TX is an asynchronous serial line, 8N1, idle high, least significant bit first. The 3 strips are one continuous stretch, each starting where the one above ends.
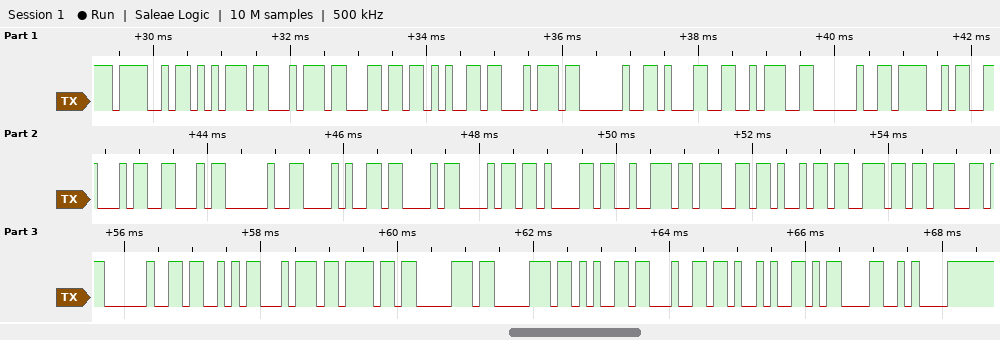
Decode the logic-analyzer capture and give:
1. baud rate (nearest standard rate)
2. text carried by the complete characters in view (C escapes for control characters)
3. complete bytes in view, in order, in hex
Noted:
9600 baud
"Outlet 1: OFF (Charging Stopped)\r\n"
0x4F 0x75 0x74 0x6C 0x65 0x74 0x20 0x31 0x3A 0x20 0x4F 0x46 0x46 0x20 0x28 0x43 0x68 0x61 0x72 0x67 0x69 0x6E 0x67 0x20 0x53 0x74 0x6F 0x70 0x70 0x65 0x64 0x29 0x0D 0x0A
